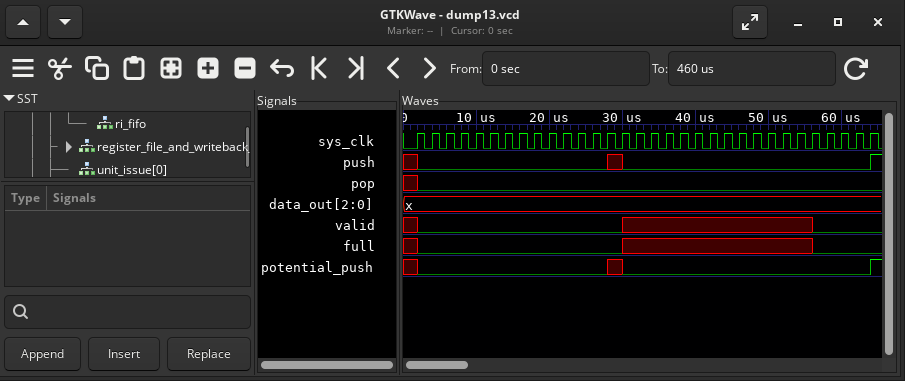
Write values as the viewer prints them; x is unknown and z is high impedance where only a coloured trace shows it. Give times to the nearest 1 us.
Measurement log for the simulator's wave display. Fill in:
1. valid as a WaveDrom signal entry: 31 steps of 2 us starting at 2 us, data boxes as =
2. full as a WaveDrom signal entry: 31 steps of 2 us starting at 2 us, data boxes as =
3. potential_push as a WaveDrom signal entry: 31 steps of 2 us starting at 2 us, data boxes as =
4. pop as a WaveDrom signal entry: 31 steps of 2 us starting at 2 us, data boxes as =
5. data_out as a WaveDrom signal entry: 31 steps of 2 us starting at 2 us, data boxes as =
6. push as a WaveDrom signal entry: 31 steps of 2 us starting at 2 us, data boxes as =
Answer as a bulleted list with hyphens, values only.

- {name: 'valid', wave: '0.............x............0...'}
- {name: 'full', wave: '0.............x............0...'}
- {name: 'potential_push', wave: '0............x0................'}
- {name: 'pop', wave: '0..............................'}
- {name: 'data_out', wave: 'x..............................'}
- {name: 'push', wave: '0............x0................'}
